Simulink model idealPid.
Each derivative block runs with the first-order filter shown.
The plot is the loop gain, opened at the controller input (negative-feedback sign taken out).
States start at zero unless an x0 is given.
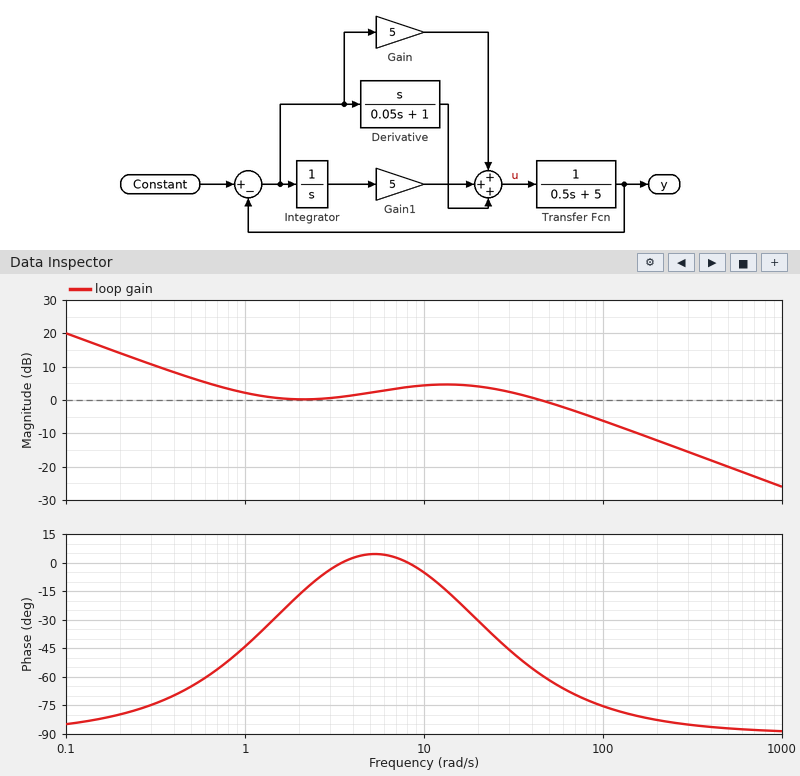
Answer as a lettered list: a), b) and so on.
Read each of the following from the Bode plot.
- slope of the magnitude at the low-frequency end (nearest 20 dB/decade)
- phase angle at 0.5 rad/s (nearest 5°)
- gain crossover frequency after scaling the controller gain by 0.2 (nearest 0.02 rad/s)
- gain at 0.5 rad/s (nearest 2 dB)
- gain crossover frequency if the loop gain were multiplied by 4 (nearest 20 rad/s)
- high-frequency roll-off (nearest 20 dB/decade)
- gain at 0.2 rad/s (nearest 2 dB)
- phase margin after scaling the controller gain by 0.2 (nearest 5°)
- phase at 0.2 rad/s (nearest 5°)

a) -20 dB/decade
b) -65°
c) 0.20 rad/s
d) 6 dB
e) 200 rad/s
f) -20 dB/decade
g) 14 dB
h) 100°
i) -80°
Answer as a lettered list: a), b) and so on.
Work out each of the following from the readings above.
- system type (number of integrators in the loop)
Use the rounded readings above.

a) 1
